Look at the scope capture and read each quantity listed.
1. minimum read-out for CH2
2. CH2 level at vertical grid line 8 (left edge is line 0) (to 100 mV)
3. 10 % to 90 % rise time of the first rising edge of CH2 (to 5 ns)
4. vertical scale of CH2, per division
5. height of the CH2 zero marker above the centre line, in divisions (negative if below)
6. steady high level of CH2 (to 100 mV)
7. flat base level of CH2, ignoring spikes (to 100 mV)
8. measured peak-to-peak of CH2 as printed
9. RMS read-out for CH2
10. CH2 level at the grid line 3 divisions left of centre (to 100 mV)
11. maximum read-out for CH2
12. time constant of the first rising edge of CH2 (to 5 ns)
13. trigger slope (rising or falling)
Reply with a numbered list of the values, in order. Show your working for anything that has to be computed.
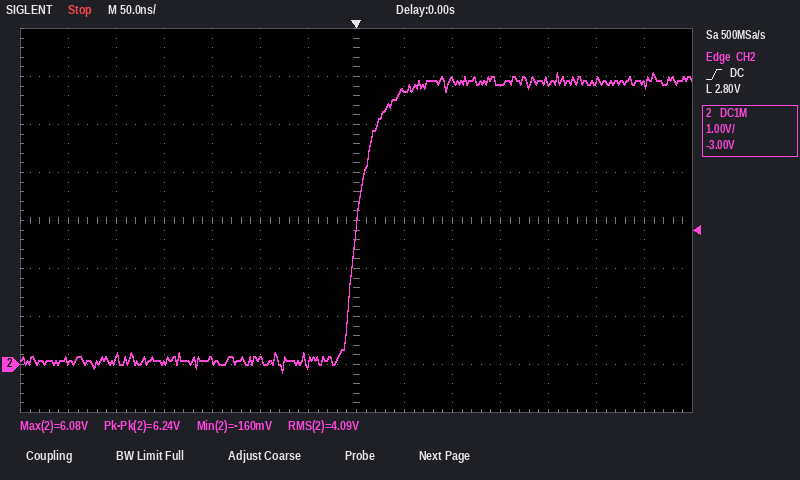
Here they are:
1. -160 mV
2. 5.7 V
3. 40 ns
4. 1 V
5. -3.0 div
6. 5.9 V
7. 100 mV
8. 6.24 V
9. 4.09 V
10. 100 mV
11. 6.08 V
12. 40 ns / 2.2 ≈ 18.2 ns, so 20 ns to the nearest 5 ns
13. rising
